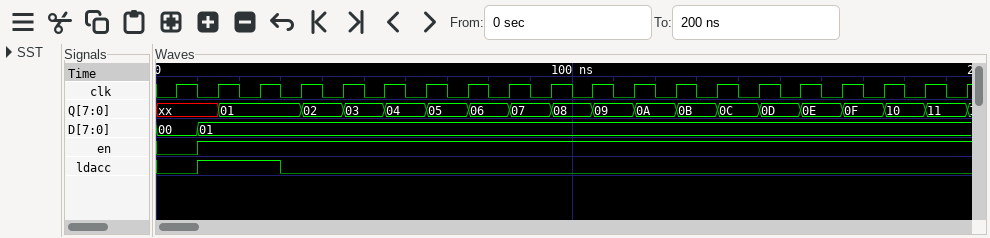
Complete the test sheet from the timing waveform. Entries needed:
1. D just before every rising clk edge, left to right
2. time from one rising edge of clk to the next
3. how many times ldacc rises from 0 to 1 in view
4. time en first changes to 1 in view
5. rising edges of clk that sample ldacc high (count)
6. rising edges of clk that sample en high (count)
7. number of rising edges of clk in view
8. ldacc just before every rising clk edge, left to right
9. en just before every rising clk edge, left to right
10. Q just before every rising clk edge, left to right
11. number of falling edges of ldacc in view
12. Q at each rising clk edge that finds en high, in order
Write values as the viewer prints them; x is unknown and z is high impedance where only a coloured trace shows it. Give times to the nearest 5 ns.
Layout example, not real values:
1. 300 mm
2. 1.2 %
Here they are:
1. 00, 01, 01, 01, 01, 01, 01, 01, 01, 01, 01, 01, 01, 01, 01, 01, 01, 01, 01, 01
2. 10 ns
3. 1
4. 10 ns
5. 2
6. 19
7. 20
8. 0 1 1 0 0 0 0 0 0 0 0 0 0 0 0 0 0 0 0 0
9. 0 1 1 1 1 1 1 1 1 1 1 1 1 1 1 1 1 1 1 1
10. xx, xx, 01, 01, 02, 03, 04, 05, 06, 07, 08, 09, 0A, 0B, 0C, 0D, 0E, 0F, 10, 11
11. 1
12. xx, 01, 01, 02, 03, 04, 05, 06, 07, 08, 09, 0A, 0B, 0C, 0D, 0E, 0F, 10, 11
